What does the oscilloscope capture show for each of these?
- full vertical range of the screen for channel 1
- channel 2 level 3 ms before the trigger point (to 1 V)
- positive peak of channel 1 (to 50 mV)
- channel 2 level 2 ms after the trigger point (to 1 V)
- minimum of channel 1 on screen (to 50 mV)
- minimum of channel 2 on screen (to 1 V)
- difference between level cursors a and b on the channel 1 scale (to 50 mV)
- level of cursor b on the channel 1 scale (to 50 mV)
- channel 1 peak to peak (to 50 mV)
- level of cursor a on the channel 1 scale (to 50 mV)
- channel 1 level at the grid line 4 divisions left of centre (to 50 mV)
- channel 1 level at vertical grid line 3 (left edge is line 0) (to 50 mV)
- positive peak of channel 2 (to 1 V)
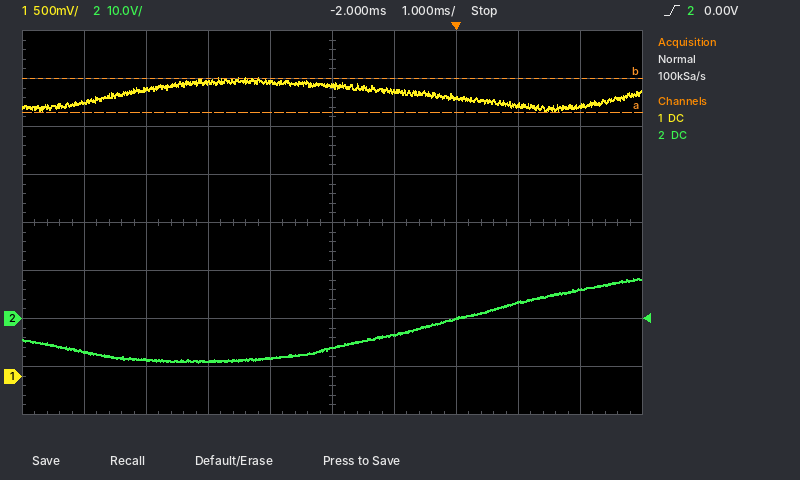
4 V
-8 V
3.10 V
6 V
2.75 V
-9 V
350 mV
3.10 V
350 mV
2.75 V
2.85 V
3.05 V
8 V
